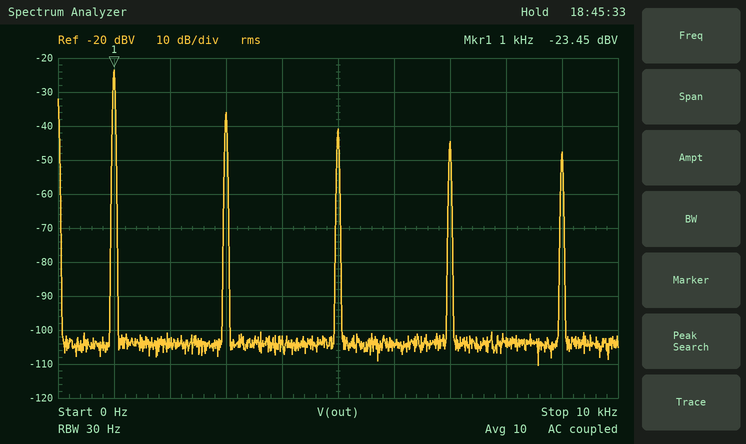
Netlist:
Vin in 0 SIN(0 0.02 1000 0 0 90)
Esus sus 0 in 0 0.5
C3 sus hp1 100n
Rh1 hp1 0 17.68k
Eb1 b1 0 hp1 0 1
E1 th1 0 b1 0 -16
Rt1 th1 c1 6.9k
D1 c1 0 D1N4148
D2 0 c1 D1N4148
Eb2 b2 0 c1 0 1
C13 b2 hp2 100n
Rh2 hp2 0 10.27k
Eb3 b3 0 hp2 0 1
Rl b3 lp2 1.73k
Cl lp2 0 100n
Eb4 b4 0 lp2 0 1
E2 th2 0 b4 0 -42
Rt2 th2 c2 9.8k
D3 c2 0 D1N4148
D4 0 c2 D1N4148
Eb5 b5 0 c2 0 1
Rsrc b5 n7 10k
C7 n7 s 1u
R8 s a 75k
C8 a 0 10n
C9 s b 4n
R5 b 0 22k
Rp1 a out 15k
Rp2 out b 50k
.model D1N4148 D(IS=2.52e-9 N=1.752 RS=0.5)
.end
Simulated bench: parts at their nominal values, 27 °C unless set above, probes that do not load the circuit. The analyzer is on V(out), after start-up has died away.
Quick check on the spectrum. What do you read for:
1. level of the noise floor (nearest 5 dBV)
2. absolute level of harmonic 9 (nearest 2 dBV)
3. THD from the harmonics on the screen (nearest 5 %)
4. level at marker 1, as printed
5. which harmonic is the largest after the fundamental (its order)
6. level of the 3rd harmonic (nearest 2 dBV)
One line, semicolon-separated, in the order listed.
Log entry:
-105 dBV; -48 dBV; 30 %; -23.45 dBV; 3; -36 dBV
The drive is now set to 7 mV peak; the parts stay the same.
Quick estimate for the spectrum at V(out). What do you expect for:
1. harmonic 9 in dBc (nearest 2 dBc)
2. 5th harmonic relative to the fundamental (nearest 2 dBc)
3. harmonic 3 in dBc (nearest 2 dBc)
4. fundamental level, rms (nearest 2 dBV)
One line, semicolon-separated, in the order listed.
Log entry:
-34 dBc; -20 dBc; -14 dBc; -24 dBV
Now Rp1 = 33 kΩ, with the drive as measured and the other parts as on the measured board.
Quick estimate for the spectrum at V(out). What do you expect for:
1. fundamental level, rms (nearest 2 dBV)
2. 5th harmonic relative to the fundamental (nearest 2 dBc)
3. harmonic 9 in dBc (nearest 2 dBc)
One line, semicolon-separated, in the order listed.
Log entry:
-24 dBV; -12 dBc; -18 dBc
